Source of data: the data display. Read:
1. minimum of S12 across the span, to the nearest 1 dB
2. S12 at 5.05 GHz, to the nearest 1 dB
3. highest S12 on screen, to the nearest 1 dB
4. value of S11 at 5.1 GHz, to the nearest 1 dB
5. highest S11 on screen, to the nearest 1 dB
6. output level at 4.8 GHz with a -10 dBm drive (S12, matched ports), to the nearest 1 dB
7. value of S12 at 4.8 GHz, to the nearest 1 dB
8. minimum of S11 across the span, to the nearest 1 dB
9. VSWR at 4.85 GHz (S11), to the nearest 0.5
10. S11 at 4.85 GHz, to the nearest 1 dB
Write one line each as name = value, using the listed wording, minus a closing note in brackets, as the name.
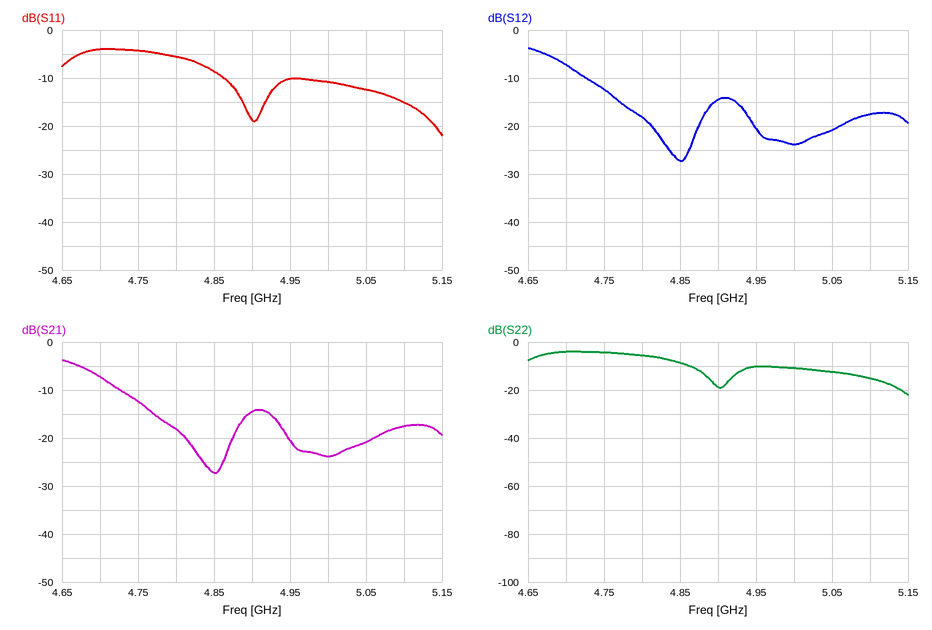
minimum of S12 across the span, to the nearest 1 dB = -27 dB
S12 at 5.05 GHz, to the nearest 1 dB = -21 dB
highest S12 on screen, to the nearest 1 dB = -4 dB
value of S11 at 5.1 GHz, to the nearest 1 dB = -15 dB
highest S11 on screen, to the nearest 1 dB = -4 dB
output level at 4.8 GHz with a -10 dBm drive (S12, matched ports), to the nearest 1 dB = -28 dBm
value of S12 at 4.8 GHz, to the nearest 1 dB = -18 dB
minimum of S11 across the span, to the nearest 1 dB = -22 dB
VSWR at 4.85 GHz (S11), to the nearest 0.5 = 2.0
S11 at 4.85 GHz, to the nearest 1 dB = -9 dB
